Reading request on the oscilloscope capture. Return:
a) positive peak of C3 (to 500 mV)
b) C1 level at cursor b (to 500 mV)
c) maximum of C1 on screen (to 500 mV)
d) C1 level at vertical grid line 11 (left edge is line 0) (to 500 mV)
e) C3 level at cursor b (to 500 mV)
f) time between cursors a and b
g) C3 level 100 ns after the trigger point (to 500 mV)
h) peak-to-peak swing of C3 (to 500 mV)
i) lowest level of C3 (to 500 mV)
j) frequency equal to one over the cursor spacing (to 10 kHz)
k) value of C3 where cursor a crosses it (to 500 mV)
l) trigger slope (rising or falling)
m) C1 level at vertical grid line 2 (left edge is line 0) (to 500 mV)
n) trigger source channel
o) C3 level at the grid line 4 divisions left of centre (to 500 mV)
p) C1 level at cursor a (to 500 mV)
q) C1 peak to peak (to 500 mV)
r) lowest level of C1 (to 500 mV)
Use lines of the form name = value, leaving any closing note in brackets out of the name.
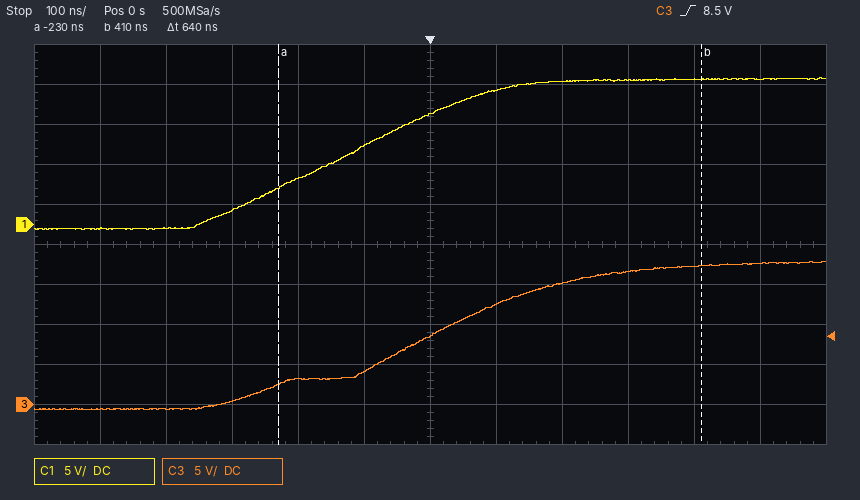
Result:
positive peak of C3 = 18.0 V
C1 level at cursor b = 18.0 V
maximum of C1 on screen = 18.5 V
C1 level at vertical grid line 11 (left edge is line 0) = 18.0 V
C3 level at cursor b = 17.5 V
time between cursors a and b = 640 ns
C3 level 100 ns after the trigger point = 12.5 V
peak-to-peak swing of C3 = 18.5 V
lowest level of C3 = -500 mV
frequency equal to one over the cursor spacing = 1.56 MHz
value of C3 where cursor a crosses it = 2.5 V
trigger slope = rising
C1 level at vertical grid line 2 (left edge is line 0) = -500 mV
trigger source channel = C3
C3 level at the grid line 4 divisions left of centre = -500 mV
C1 level at cursor a = 4.5 V
C1 peak to peak = 19.0 V
lowest level of C1 = -500 mV
